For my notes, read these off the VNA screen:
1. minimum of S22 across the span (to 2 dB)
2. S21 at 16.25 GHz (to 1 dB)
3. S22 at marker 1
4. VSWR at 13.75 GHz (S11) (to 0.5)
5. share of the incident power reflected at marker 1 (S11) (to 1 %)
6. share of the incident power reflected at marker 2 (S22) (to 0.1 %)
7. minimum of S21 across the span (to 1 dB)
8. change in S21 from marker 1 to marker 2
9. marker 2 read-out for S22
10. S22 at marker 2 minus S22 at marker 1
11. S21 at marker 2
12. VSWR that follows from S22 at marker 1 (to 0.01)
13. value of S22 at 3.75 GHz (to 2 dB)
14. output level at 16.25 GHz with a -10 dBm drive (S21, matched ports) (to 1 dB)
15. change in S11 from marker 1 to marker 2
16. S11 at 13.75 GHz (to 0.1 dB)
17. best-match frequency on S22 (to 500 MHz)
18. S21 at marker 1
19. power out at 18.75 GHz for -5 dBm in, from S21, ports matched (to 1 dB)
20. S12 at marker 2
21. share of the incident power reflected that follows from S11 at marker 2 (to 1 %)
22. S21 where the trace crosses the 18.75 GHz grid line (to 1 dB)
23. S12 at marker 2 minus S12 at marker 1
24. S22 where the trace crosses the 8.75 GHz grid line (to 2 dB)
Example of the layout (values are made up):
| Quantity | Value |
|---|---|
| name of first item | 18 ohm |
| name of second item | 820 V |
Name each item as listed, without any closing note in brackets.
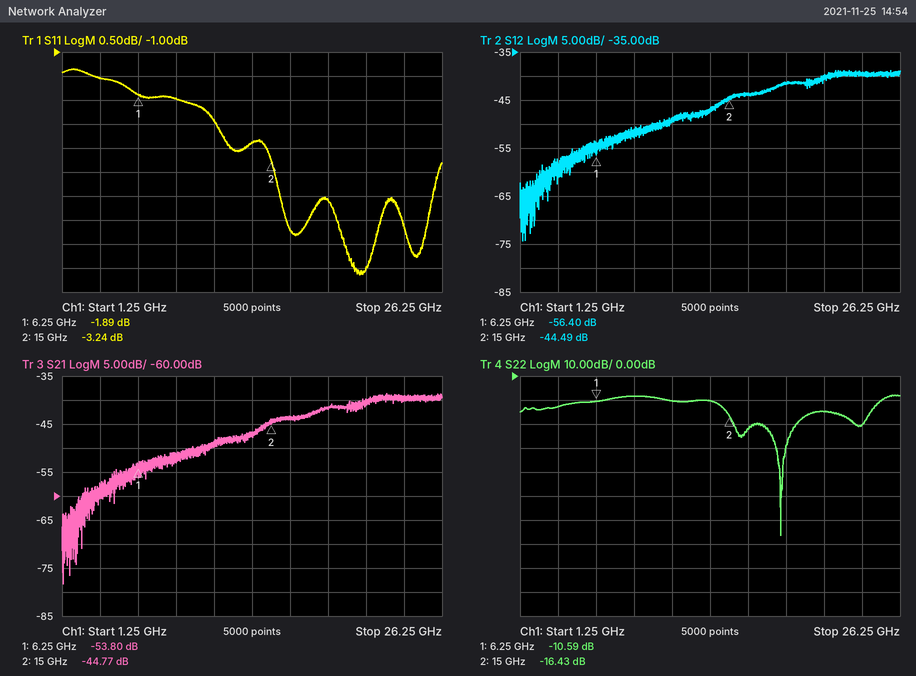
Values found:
| Quantity | Value |
|---|---|
| minimum of S22 across the span | -66 dB |
| S21 at 16.25 GHz | -44 dB |
| S22 at marker 1 | -10.59 dB |
| VSWR at 13.75 GHz (S11) | 6.0 |
| share of the incident power reflected at marker 1 (S11) | 65 % |
| share of the incident power reflected at marker 2 (S22) | 2.3 % |
| minimum of S21 across the span | -78 dB |
| change in S21 from marker 1 to marker 2 | 9.03 dB |
| marker 2 read-out for S22 | -16.43 dB |
| S22 at marker 2 minus S22 at marker 1 | -5.84 dB |
| S21 at marker 2 | -44.77 dB |
| VSWR that follows from S22 at marker 1 | 1.84 |
| value of S22 at 3.75 GHz | -12 dB |
| output level at 16.25 GHz with a -10 dBm drive (S21, matched ports) | -54 dBm |
| change in S11 from marker 1 to marker 2 | -1.35 dB |
| S11 at 13.75 GHz | -2.9 dB |
| best-match frequency on S22 | 18.5 GHz |
| S21 at marker 1 | -53.80 dB |
| power out at 18.75 GHz for -5 dBm in, from S21, ports matched | -47 dBm |
| S12 at marker 2 | -44.49 dB |
| share of the incident power reflected that follows from S11 at marker 2 | 47 % |
| S21 where the trace crosses the 18.75 GHz grid line | -42 dB |
| S12 at marker 2 minus S12 at marker 1 | 11.91 dB |
| S22 where the trace crosses the 8.75 GHz grid line | -8 dB |
